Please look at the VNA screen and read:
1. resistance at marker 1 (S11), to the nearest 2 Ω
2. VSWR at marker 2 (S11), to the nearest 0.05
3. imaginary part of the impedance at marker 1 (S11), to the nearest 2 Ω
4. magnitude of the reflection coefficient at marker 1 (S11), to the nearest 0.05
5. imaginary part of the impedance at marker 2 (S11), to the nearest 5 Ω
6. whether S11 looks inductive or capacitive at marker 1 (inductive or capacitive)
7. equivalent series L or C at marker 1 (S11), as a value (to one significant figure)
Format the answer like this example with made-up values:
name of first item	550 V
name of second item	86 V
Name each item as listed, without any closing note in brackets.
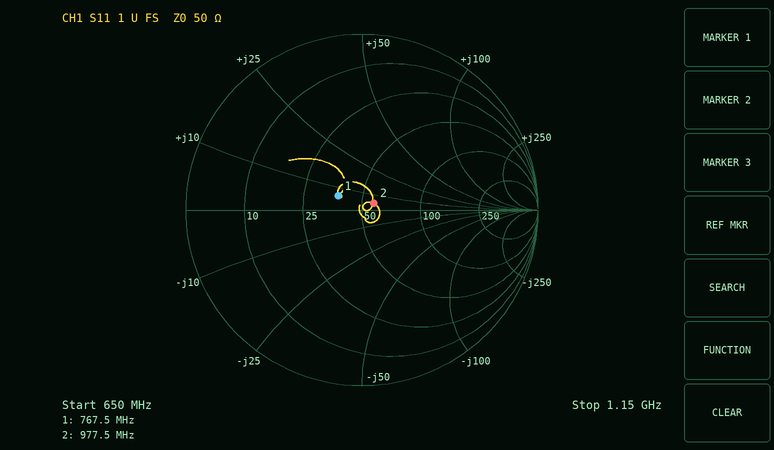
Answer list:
resistance at marker 1 (S11), to the nearest 2 Ω	38 Ω
VSWR at marker 2 (S11), to the nearest 0.05	1.15
imaginary part of the impedance at marker 1 (S11), to the nearest 2 Ω	+6 Ω
magnitude of the reflection coefficient at marker 1 (S11), to the nearest 0.05	0.15
imaginary part of the impedance at marker 2 (S11), to the nearest 5 Ω	+5 Ω
whether S11 looks inductive or capacitive at marker 1	inductive
equivalent series L or C at marker 1 (S11), as a value	1 nH
